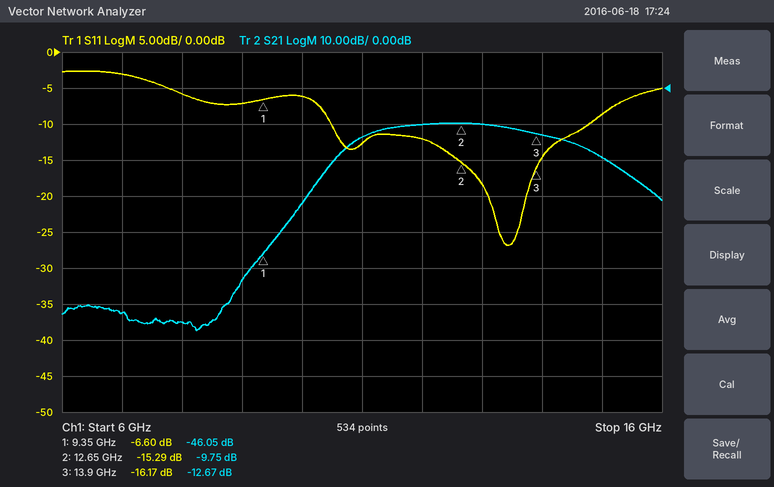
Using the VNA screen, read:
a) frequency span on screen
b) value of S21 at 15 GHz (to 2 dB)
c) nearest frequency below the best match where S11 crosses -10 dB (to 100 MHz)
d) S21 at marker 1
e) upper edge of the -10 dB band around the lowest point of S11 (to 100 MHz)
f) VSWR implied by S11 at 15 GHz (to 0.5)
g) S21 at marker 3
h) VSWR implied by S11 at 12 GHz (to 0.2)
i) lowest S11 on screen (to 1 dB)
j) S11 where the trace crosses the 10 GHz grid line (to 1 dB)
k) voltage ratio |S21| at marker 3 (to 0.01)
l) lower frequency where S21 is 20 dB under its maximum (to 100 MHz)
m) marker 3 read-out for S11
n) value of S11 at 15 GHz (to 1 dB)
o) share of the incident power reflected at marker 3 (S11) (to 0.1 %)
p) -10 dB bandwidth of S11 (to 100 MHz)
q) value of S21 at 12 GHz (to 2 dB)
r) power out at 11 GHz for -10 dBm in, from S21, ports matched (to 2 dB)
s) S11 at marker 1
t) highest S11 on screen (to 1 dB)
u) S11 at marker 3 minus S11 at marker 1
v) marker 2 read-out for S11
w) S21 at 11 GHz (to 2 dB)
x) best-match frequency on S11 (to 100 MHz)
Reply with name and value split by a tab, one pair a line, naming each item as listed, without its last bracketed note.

frequency span on screen	10 GHz
value of S21 at 15 GHz	-20 dB
nearest frequency below the best match where S11 crosses -10 dB	10.5 GHz
S21 at marker 1	-46.05 dB
upper edge of the -10 dB band around the lowest point of S11	14.8 GHz
VSWR implied by S11 at 15 GHz	2.0
S21 at marker 3	-12.67 dB
VSWR implied by S11 at 12 GHz	1.6
lowest S11 on screen	-27 dB
S11 where the trace crosses the 10 GHz grid line	-6 dB
voltage ratio |S21| at marker 3	0.23
lower frequency where S21 is 20 dB under its maximum	10.1 GHz
marker 3 read-out for S11	-16.17 dB
value of S11 at 15 GHz	-9 dB
share of the incident power reflected at marker 3 (S11)	2.4 %
-10 dB bandwidth of S11	4.3 GHz
value of S21 at 12 GHz	-10 dB
power out at 11 GHz for -10 dBm in, from S21, ports matched	-24 dBm
S11 at marker 1	-6.60 dB
highest S11 on screen	-3 dB
S11 at marker 3 minus S11 at marker 1	-9.57 dB
marker 2 read-out for S11	-15.29 dB
S21 at 11 GHz	-14 dB
best-match frequency on S11	13.4 GHz
